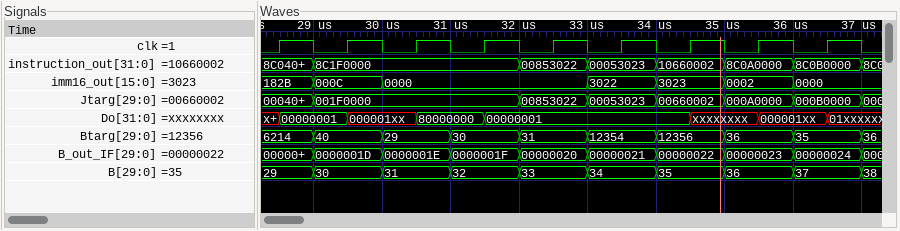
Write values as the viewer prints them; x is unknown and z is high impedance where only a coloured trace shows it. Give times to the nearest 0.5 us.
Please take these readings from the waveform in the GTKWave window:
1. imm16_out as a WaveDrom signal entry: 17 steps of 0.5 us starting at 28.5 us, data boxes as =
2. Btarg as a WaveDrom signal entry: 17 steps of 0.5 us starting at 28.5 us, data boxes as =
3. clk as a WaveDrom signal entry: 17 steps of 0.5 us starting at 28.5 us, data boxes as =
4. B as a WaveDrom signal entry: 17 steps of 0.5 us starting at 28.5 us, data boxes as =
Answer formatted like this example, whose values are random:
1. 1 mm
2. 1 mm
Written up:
1. {name: 'imm16_out', wave: '==.=.....=.=.=.=.', data: '182B 000C 0000 3022 3023 0002 0000'}
2. {name: 'Btarg', wave: '==.=.=.=.=.=.=.=.', data: '6214 40 29 30 31 12354 12356 36 35'}
3. {name: 'clk', wave: '10101010101010101'}
4. {name: 'B', wave: '==.=.=.=.=.=.=.=.', data: '29 30 31 32 33 34 35 36 37'}
